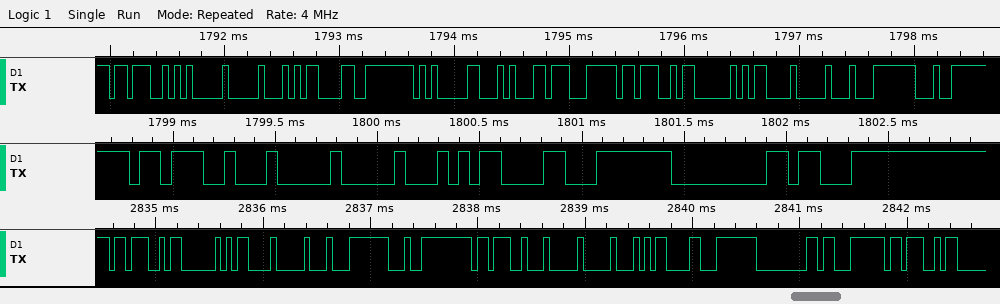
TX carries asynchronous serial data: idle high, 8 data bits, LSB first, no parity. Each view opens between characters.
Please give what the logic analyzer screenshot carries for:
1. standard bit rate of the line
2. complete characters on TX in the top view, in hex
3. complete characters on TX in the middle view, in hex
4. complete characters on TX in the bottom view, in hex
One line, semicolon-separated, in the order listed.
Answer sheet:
19200 baud; 3B, 05, 10, 0D, FE, 05, 14, C7, 3B, 03, 0D, 10, FC, E4; 3B, 04, 10, 0D, FC, 00, E3; 3B, 03, 0D, 10, FC, E4, 3B, 04, 10, 0D, FC, 00, E3, 3B
